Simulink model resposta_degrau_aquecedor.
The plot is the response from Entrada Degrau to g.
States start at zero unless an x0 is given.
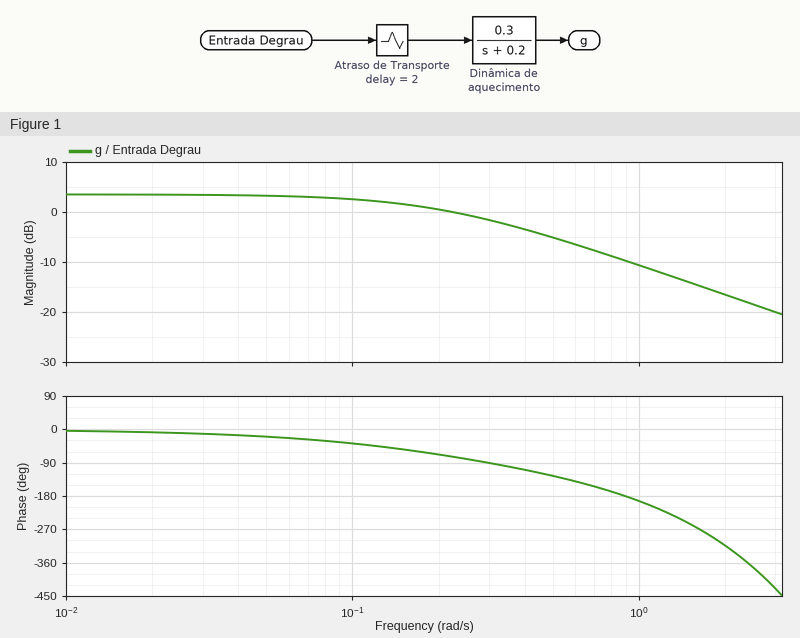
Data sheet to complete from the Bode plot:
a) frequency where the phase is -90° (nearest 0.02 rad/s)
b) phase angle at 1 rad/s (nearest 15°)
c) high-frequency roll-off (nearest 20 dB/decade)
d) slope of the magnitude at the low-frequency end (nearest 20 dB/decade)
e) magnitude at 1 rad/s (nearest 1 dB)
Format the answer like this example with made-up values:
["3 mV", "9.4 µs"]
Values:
["0.30 rad/s", "-195°", "-20 dB/decade", "0 dB/decade", "-11 dB"]
